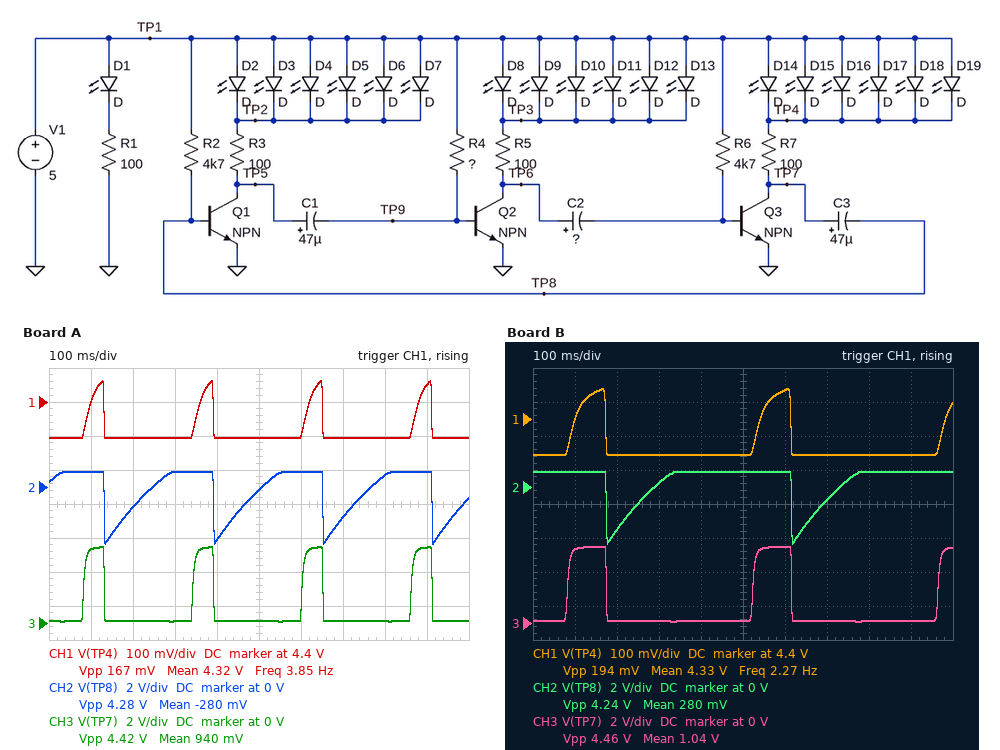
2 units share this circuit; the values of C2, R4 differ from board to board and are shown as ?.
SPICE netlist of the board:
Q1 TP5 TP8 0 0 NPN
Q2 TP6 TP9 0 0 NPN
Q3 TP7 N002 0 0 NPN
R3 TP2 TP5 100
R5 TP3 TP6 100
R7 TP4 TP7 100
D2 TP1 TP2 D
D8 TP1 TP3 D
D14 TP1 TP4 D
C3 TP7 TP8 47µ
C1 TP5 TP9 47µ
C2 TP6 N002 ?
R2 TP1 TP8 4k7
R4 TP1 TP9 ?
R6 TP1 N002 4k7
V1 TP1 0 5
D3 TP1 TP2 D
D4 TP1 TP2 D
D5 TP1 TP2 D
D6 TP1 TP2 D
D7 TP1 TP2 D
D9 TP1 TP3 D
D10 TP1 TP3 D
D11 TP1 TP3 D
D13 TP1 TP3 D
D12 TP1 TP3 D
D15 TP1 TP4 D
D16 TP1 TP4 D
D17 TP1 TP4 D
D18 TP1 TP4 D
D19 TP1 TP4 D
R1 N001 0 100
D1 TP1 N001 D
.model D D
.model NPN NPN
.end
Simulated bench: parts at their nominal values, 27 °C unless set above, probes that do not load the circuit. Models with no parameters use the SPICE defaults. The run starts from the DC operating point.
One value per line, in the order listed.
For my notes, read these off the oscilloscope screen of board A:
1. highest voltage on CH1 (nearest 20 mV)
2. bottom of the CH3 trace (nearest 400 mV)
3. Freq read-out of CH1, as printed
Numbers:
4.46 V
0 V
3.85 Hz
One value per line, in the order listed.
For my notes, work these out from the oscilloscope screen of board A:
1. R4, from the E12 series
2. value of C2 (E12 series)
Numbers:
1.5 kΩ
15 µF
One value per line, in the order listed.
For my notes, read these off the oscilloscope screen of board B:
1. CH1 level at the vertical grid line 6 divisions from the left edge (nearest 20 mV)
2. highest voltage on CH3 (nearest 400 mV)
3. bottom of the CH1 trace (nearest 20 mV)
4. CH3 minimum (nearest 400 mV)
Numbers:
4.48 V
4.4 V
4.30 V
0 V
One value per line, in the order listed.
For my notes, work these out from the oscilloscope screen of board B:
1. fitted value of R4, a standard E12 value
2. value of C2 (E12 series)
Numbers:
5.6 kΩ
27 µF
